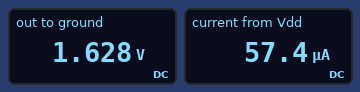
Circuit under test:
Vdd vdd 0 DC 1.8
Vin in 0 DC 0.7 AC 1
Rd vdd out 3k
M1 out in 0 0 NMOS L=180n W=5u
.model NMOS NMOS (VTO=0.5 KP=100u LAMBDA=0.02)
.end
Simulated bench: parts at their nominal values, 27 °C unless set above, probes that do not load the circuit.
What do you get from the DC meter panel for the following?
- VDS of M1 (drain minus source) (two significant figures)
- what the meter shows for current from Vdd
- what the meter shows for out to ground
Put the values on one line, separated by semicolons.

1.6 V; 57.4 µA; 1.628 V
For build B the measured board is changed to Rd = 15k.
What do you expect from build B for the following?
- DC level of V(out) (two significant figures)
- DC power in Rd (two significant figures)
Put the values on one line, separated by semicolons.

950 mV; 48 µW
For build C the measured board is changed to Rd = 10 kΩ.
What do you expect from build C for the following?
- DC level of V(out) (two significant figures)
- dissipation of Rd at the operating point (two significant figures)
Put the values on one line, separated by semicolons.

1.2 V; 32 µW
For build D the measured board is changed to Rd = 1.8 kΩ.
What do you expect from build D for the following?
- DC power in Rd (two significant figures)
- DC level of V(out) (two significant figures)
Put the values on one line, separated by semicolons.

5.9 µW; 1.7 V
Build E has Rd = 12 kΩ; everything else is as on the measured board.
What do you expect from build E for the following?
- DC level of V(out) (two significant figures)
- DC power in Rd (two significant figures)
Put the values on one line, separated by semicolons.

1.1 V; 39 µW
